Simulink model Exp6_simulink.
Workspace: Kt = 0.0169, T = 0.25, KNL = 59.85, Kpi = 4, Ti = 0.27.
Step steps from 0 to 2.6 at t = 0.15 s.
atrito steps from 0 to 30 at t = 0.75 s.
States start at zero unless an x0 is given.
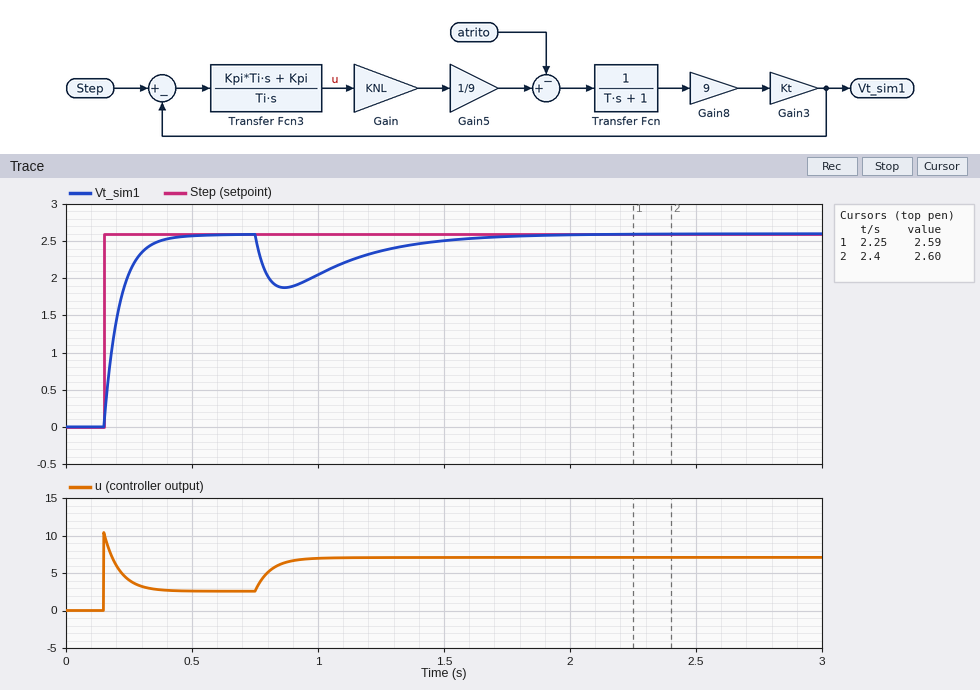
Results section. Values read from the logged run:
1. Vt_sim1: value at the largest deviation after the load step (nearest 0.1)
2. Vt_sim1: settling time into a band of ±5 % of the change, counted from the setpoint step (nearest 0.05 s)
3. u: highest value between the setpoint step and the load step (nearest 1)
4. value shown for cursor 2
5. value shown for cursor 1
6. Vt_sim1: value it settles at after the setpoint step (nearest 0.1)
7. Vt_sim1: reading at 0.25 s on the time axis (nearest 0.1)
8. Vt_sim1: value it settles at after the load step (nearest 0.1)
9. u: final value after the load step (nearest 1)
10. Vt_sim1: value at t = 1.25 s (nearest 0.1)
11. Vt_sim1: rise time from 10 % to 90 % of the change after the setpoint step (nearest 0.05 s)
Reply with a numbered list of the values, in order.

1. 1.9
2. 0.20 s
3. 10
4. 2.60
5. 2.59
6. 2.6
7. 2.1
8. 2.6
9. 7
10. 2.4
11. 0.15 s
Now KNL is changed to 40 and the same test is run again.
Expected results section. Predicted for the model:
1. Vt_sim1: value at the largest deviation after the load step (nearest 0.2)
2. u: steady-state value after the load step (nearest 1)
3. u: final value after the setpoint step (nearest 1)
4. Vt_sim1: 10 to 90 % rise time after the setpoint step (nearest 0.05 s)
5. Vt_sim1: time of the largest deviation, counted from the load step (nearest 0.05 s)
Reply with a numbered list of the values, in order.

1. 1.6
2. 11
3. 4
4. 0.20 s
5. 0.15 s
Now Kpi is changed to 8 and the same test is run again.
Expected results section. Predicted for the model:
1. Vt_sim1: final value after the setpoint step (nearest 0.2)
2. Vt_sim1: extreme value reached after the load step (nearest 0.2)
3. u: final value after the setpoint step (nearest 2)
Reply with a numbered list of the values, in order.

1. 2.6
2. 2.2
3. 2
